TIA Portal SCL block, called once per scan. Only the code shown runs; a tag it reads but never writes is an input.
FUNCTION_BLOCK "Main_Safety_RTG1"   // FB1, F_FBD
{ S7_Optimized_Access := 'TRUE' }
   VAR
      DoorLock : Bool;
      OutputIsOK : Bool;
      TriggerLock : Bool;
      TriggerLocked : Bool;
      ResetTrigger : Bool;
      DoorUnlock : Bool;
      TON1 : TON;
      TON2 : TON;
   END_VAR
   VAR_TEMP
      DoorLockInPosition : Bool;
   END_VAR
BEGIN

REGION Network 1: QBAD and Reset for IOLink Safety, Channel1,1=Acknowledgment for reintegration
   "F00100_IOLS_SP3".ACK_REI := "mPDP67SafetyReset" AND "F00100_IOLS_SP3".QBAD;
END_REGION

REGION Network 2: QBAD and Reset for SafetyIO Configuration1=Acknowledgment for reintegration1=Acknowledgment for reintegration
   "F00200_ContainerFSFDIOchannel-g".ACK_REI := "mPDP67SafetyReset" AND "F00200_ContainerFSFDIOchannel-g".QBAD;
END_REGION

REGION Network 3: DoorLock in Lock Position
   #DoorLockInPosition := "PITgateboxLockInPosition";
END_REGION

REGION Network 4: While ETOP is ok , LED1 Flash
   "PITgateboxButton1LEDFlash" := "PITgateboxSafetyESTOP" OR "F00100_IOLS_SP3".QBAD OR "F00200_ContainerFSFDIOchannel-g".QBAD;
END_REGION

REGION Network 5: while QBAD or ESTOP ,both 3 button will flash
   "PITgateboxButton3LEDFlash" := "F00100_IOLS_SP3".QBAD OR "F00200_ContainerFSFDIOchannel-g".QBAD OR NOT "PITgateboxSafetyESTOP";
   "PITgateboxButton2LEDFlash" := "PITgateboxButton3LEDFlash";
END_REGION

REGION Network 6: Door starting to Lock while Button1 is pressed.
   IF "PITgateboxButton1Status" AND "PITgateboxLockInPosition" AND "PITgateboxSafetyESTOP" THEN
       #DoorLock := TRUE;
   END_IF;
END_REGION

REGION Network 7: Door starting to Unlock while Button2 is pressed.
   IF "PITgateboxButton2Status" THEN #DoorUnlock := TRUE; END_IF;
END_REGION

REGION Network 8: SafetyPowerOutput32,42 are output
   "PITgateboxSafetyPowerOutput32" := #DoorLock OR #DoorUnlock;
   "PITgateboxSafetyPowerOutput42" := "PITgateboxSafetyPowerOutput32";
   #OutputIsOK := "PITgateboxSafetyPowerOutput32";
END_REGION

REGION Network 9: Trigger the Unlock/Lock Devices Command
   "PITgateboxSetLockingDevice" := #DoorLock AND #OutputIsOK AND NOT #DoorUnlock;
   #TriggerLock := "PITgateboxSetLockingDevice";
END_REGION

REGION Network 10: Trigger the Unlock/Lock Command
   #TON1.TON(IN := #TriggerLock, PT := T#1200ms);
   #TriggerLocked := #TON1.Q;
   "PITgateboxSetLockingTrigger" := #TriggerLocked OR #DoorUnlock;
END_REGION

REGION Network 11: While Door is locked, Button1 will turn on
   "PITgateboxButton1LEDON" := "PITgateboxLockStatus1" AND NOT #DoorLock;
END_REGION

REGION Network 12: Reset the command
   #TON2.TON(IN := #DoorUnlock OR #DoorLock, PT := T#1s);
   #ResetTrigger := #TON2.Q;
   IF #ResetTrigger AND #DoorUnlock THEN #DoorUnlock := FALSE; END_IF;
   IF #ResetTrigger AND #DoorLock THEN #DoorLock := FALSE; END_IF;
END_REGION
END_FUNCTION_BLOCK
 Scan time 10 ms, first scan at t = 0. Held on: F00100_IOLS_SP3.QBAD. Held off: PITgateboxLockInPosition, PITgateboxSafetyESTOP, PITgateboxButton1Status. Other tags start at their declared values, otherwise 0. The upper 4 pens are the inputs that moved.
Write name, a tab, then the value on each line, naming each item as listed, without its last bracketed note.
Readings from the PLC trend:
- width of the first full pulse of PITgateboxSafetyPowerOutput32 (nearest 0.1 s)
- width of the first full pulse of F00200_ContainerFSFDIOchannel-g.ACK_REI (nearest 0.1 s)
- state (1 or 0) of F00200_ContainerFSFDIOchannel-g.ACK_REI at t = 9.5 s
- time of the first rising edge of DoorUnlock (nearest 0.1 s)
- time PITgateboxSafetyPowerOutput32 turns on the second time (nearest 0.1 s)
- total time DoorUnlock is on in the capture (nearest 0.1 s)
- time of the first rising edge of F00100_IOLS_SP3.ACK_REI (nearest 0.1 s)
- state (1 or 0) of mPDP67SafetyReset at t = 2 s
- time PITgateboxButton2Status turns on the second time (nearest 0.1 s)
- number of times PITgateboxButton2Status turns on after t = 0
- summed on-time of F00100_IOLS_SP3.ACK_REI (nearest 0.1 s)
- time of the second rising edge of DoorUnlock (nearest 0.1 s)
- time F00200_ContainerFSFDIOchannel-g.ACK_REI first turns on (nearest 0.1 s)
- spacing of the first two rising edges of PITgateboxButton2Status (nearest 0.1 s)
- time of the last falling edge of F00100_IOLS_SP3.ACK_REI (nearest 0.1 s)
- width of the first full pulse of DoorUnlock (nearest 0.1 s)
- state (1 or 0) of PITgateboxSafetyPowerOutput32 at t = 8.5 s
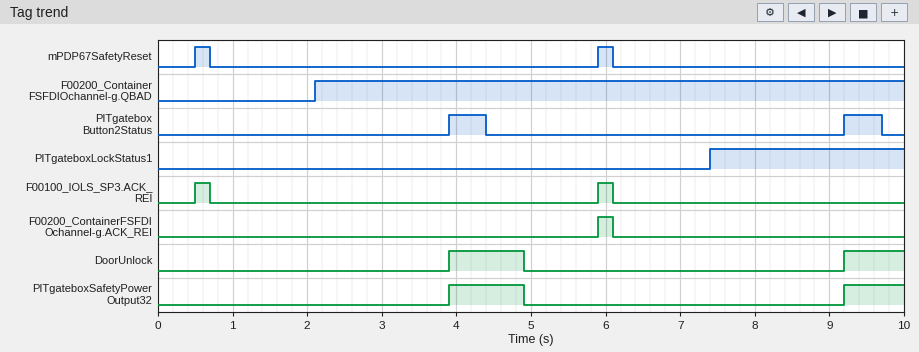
width of the first full pulse of PITgateboxSafetyPowerOutput32	1.0 s
width of the first full pulse of F00200_ContainerFSFDIOchannel-g.ACK_REI	0.2 s
state (1 or 0) of F00200_ContainerFSFDIOchannel-g.ACK_REI at t = 9.5 s	0
time of the first rising edge of DoorUnlock	3.9 s
time PITgateboxSafetyPowerOutput32 turns on the second time	9.2 s
total time DoorUnlock is on in the capture	1.8 s
time of the first rising edge of F00100_IOLS_SP3.ACK_REI	0.5 s
state (1 or 0) of mPDP67SafetyReset at t = 2 s	0
time PITgateboxButton2Status turns on the second time	9.2 s
number of times PITgateboxButton2Status turns on after t = 0	2
summed on-time of F00100_IOLS_SP3.ACK_REI	0.4 s
time of the second rising edge of DoorUnlock	9.2 s
time F00200_ContainerFSFDIOchannel-g.ACK_REI first turns on	5.9 s
spacing of the first two rising edges of PITgateboxButton2Status	5.3 s
time of the last falling edge of F00100_IOLS_SP3.ACK_REI	6.1 s
width of the first full pulse of DoorUnlock	1.0 s
state (1 or 0) of PITgateboxSafetyPowerOutput32 at t = 8.5 s	0
